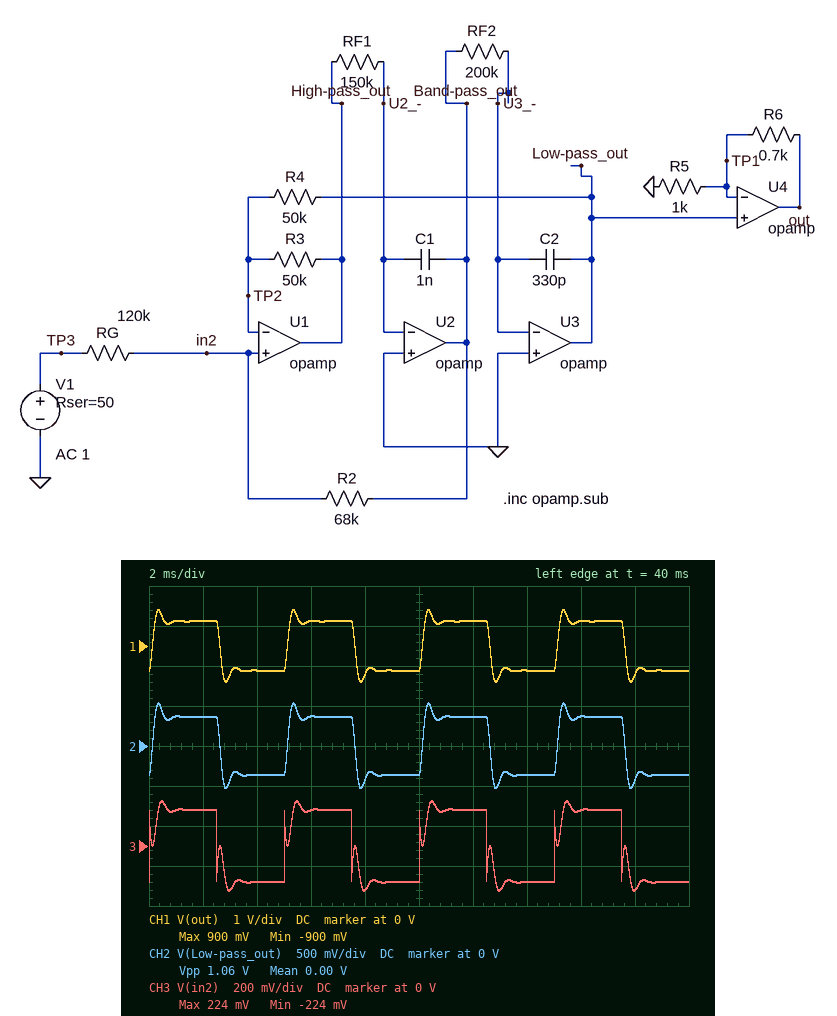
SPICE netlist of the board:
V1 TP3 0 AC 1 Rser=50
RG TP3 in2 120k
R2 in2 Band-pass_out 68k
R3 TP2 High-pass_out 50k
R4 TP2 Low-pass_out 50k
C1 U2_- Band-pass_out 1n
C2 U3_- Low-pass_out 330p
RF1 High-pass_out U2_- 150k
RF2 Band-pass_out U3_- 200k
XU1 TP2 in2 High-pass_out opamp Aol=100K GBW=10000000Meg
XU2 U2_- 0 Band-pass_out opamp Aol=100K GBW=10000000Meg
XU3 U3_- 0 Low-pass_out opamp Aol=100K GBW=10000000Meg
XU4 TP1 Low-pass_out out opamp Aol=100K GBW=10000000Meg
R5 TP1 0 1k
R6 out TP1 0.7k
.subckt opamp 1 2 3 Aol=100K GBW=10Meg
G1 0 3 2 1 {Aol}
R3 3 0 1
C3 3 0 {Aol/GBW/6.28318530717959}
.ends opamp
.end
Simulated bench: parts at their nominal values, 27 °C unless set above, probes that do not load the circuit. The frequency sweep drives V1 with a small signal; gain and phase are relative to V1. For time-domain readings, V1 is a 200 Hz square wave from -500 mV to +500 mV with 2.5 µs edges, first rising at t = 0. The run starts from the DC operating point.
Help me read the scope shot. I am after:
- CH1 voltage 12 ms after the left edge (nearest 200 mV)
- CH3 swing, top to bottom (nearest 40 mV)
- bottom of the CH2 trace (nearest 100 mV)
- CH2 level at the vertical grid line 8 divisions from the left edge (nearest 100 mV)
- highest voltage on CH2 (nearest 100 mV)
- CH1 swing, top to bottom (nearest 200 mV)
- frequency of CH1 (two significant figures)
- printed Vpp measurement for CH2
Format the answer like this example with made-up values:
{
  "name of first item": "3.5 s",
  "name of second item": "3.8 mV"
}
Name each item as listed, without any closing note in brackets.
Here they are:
{
  "CH1 voltage 12 ms after the left edge": "600 mV",
  "CH3 swing, top to bottom": "440 mV",
  "bottom of the CH2 trace": "-500 mV",
  "CH2 level at the vertical grid line 8 divisions from the left edge": "400 mV",
  "highest voltage on CH2": "500 mV",
  "CH1 swing, top to bottom": "1.8 V",
  "frequency of CH1": "200 Hz",
  "printed Vpp measurement for CH2": "1.06 V"
}
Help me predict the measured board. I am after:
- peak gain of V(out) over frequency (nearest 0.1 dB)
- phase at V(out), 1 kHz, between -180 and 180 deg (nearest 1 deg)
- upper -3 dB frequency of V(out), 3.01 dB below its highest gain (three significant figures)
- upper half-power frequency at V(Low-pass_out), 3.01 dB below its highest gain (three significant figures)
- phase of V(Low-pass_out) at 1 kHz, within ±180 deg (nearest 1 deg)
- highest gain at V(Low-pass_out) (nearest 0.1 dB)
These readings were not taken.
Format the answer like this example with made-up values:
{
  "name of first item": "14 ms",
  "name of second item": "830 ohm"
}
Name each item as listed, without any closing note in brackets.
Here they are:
{
  "peak gain of V(out) over frequency": "4.1 dB",
  "phase at V(out), 1 kHz, between -180 and 180 deg": "-41 deg",
  "upper -3 dB frequency of V(out), 3.01 dB below its highest gain": "1.90 kHz",
  "upper half-power frequency at V(Low-pass_out), 3.01 dB below its highest gain": "1.90 kHz",
  "phase of V(Low-pass_out) at 1 kHz, within ±180 deg": "-41 deg",
  "highest gain at V(Low-pass_out)": "-0.5 dB"
}
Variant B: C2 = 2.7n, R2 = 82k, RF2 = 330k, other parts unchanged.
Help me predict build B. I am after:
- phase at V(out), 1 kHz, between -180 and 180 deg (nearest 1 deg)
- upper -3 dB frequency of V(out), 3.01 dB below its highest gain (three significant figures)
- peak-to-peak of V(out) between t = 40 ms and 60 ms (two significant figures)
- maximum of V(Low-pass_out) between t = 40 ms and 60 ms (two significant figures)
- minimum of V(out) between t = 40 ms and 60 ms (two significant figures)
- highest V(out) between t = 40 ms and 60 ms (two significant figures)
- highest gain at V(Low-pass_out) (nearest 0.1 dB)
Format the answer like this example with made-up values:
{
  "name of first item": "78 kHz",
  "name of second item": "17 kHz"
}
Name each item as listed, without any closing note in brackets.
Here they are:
{
  "phase at V(out), 1 kHz, between -180 and 180 deg": "-123 deg",
  "upper -3 dB frequency of V(out), 3.01 dB below its highest gain": "170 Hz",
  "peak-to-peak of V(out) between t = 40 ms and 60 ms": "1.2 V",
  "maximum of V(Low-pass_out) between t = 40 ms and 60 ms": "350 mV",
  "minimum of V(out) between t = 40 ms and 60 ms": "-590 mV",
  "highest V(out) between t = 40 ms and 60 ms": "590 mV",
  "highest gain at V(Low-pass_out)": "-1.8 dB"
}
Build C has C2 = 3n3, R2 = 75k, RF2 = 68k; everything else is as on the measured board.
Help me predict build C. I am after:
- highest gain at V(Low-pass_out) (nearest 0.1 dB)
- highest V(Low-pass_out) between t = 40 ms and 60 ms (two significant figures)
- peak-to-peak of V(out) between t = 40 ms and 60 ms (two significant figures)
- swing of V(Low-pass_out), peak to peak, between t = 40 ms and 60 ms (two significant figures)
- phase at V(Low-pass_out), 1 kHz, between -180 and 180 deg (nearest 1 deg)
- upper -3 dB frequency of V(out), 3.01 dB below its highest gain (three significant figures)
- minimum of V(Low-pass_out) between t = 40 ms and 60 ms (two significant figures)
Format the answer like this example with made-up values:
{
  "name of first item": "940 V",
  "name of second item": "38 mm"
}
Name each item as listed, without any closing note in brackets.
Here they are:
{
  "highest gain at V(Low-pass_out)": "-2.3 dB",
  "highest V(Low-pass_out) between t = 40 ms and 60 ms": "410 mV",
  "peak-to-peak of V(out) between t = 40 ms and 60 ms": "1.4 V",
  "swing of V(Low-pass_out), peak to peak, between t = 40 ms and 60 ms": "810 mV",
  "phase at V(Low-pass_out), 1 kHz, between -180 and 180 deg": "-101 deg",
  "upper -3 dB frequency of V(out), 3.01 dB below its highest gain": "812 Hz",
  "minimum of V(Low-pass_out) between t = 40 ms and 60 ms": "-410 mV"
}
